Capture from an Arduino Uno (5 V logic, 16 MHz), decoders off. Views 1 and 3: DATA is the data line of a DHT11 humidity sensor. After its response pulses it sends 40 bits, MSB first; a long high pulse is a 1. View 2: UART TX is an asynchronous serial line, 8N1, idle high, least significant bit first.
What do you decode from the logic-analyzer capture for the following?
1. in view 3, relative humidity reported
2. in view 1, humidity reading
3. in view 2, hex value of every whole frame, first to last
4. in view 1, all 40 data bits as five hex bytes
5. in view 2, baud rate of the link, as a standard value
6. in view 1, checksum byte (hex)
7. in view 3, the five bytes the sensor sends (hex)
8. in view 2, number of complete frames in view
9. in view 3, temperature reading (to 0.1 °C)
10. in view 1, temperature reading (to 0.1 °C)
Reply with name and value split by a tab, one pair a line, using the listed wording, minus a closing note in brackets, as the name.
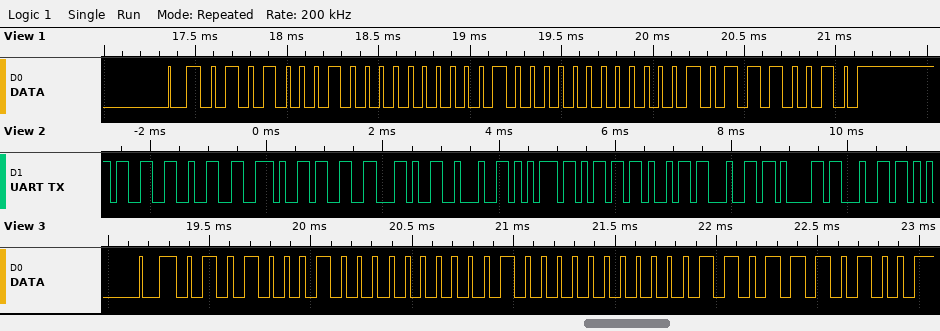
in view 3, relative humidity reported	81 %
in view 1, humidity reading	81 %
in view 2, hex value of every whole frame, first to last	33 32 2E 33 2C 22 75 6D 69 64 61 64
in view 1, all 40 data bits as five hex bytes	51 00 20 01 72
in view 2, baud rate of the link, as a standard value	9600 baud
in view 1, checksum byte	0x72
in view 3, the five bytes the sensor sends	51 00 20 03 74
in view 2, number of complete frames in view	12
in view 3, temperature reading	32.3 °C
in view 1, temperature reading	32.1 °C
